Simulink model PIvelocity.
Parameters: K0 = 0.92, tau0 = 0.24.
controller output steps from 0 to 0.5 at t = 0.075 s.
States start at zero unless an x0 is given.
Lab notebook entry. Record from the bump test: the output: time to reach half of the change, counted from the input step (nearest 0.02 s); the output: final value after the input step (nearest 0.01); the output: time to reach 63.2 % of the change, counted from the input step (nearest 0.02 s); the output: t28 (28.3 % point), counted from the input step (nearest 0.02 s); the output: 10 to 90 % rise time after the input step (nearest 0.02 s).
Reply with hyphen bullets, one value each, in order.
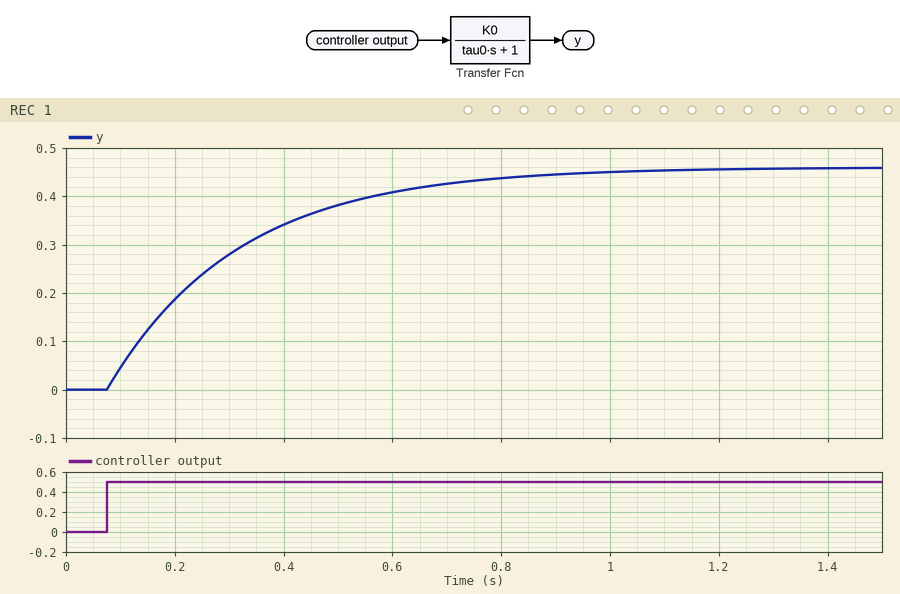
- 0.16 s
- 0.46
- 0.24 s
- 0.08 s
- 0.52 s
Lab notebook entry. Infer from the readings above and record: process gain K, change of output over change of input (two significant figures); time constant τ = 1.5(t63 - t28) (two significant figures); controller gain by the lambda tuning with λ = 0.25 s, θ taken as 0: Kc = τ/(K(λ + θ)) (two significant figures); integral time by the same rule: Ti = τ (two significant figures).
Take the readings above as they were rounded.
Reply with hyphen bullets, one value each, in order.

- 0.92
- 0.24 s
- 1.0
- 0.24 s
